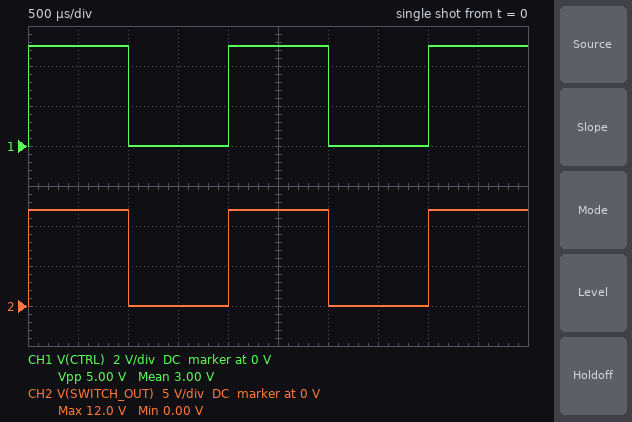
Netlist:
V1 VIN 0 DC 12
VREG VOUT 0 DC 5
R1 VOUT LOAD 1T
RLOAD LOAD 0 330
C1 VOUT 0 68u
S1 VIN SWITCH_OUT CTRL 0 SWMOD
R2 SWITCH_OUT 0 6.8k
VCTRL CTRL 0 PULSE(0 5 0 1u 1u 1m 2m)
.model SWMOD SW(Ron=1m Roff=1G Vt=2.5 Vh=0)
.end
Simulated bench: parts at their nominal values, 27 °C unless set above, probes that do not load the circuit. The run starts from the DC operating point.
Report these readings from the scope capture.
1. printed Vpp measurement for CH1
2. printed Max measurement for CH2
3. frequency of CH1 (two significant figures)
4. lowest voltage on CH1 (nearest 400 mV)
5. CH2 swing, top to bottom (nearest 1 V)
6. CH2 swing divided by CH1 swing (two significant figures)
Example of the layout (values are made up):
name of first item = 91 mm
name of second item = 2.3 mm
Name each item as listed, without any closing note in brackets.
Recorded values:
printed Vpp measurement for CH1 = 5.00 V
printed Max measurement for CH2 = 12.0 V
frequency of CH1 = 500 Hz
lowest voltage on CH1 = 0 V
CH2 swing, top to bottom = 12 V
CH2 swing divided by CH1 swing = 2.4
